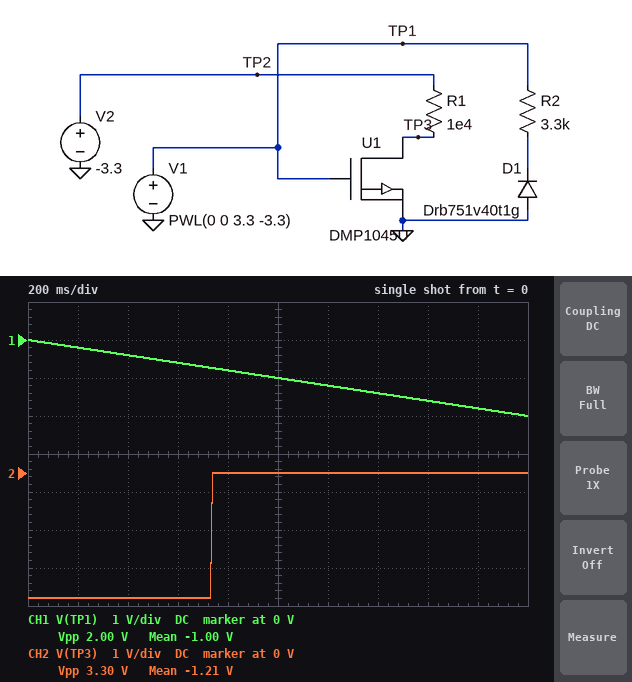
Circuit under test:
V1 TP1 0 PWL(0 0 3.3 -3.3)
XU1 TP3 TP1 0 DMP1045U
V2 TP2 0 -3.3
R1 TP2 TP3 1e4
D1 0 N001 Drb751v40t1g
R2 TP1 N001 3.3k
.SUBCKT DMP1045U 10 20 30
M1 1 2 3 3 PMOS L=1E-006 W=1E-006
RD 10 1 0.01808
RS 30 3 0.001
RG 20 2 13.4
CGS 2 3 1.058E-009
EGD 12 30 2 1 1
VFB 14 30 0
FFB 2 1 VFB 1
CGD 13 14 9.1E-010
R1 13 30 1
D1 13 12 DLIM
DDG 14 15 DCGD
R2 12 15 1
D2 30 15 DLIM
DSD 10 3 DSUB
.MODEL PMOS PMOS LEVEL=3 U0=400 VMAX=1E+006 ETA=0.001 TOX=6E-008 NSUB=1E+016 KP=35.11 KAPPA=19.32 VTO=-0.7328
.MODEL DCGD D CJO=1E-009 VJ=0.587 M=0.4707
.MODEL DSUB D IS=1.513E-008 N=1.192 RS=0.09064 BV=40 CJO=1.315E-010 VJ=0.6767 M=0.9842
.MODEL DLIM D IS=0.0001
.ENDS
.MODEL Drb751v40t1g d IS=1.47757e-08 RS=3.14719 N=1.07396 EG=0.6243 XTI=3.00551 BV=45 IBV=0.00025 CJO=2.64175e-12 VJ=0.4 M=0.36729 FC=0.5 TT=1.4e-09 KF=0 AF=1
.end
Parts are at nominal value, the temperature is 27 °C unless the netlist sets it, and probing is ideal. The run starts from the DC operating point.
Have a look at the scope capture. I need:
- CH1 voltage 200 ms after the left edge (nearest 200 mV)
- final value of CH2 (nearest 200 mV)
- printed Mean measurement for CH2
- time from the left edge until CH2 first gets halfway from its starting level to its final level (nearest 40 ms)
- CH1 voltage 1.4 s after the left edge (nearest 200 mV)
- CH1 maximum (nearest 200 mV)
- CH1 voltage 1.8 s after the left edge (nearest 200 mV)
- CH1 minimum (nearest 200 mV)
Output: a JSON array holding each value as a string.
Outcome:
["-200 mV", "0 V", "-1.21 V", "720 ms", "-1.4 V", "0 V", "-1.8 V", "-2.0 V"]
